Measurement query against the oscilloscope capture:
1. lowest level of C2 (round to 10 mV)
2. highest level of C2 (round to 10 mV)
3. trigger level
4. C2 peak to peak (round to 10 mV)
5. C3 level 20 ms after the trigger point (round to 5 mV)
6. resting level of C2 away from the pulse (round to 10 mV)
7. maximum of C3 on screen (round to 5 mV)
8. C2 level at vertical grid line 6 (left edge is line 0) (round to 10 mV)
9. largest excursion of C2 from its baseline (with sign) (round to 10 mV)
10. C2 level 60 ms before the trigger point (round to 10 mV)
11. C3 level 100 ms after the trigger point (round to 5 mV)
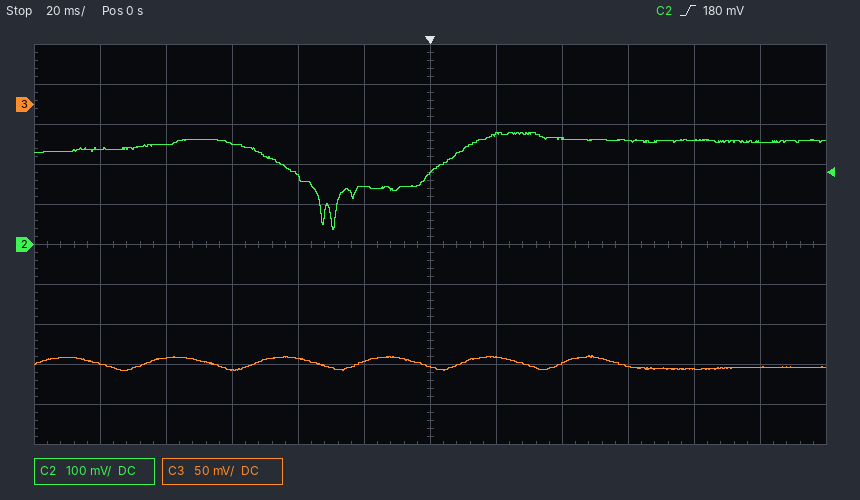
40 mV
280 mV
180 mV
240 mV
-315 mV
260 mV
-315 mV
180 mV
-220 mV
250 mV
-330 mV
